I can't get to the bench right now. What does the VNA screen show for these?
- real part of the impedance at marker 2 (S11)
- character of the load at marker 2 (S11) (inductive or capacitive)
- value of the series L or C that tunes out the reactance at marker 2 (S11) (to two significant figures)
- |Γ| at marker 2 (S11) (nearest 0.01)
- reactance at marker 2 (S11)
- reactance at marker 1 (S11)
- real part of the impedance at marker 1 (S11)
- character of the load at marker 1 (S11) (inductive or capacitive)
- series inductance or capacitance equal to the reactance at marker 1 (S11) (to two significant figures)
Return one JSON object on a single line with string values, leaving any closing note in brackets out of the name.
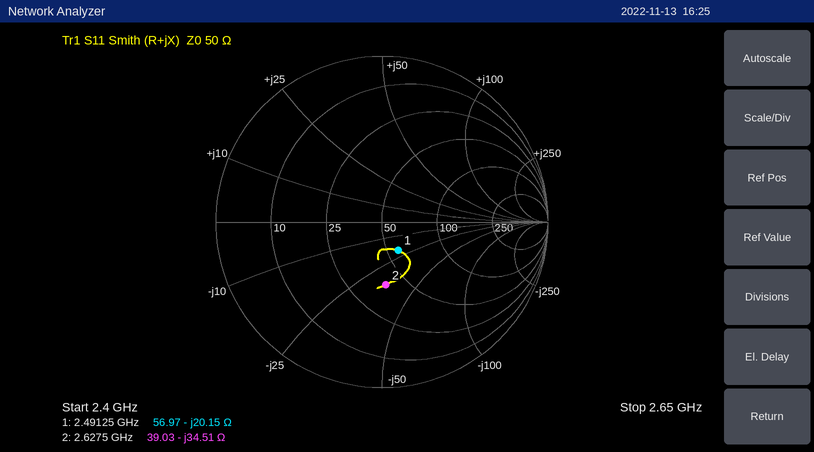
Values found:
{"real part of the impedance at marker 2": "39.03 Ω", "character of the load at marker 2 (S11)": "capacitive", "value of the series L or C that tunes out the reactance at marker 2 (S11)": "2.1 nH", "|Γ| at marker 2 (S11)": "0.38", "reactance at marker 2": "-34.51 Ω", "reactance at marker 1": "-20.15 Ω", "real part of the impedance at marker 1": "56.97 Ω", "character of the load at marker 1 (S11)": "capacitive", "series inductance or capacitance equal to the reactance at marker 1 (S11)": "3.2 pF"}
